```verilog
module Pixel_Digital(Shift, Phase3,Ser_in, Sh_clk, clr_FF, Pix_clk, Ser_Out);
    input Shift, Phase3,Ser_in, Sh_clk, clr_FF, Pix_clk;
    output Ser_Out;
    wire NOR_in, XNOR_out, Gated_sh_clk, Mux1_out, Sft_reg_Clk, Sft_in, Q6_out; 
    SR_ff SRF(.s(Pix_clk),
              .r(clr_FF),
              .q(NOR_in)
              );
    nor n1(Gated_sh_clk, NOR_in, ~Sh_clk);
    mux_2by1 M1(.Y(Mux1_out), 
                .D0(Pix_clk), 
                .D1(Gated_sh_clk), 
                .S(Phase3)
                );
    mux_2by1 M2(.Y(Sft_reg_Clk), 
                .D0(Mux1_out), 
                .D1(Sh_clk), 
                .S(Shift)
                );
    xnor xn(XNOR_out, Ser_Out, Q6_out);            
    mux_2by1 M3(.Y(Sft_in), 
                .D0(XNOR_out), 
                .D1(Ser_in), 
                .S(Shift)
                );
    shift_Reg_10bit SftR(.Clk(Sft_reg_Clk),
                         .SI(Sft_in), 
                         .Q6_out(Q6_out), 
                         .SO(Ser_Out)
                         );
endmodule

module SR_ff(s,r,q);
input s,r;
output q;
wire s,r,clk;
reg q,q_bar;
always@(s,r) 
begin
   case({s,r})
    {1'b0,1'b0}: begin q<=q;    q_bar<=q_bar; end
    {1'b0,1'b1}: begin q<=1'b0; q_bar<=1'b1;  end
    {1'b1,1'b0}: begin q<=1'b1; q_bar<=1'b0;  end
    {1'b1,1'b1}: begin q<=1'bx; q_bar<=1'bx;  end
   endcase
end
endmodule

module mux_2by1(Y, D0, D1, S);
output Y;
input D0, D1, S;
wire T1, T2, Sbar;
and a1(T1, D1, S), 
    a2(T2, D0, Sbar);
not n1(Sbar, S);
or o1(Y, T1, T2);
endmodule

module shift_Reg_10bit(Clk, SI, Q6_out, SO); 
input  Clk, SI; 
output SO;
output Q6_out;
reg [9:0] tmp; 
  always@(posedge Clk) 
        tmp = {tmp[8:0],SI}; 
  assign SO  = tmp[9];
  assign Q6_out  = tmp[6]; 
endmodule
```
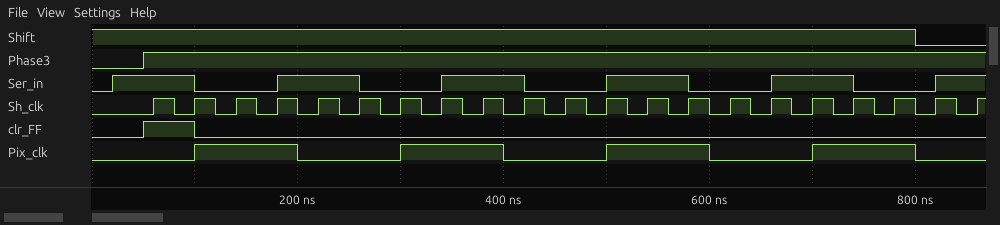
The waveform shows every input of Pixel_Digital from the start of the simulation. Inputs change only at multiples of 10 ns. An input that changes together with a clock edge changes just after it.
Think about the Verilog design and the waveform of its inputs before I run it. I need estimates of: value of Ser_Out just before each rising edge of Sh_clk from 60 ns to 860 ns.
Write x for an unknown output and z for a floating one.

x x x x x x x x x x 1 1 0 0 1 1 0 0 1 1 1
